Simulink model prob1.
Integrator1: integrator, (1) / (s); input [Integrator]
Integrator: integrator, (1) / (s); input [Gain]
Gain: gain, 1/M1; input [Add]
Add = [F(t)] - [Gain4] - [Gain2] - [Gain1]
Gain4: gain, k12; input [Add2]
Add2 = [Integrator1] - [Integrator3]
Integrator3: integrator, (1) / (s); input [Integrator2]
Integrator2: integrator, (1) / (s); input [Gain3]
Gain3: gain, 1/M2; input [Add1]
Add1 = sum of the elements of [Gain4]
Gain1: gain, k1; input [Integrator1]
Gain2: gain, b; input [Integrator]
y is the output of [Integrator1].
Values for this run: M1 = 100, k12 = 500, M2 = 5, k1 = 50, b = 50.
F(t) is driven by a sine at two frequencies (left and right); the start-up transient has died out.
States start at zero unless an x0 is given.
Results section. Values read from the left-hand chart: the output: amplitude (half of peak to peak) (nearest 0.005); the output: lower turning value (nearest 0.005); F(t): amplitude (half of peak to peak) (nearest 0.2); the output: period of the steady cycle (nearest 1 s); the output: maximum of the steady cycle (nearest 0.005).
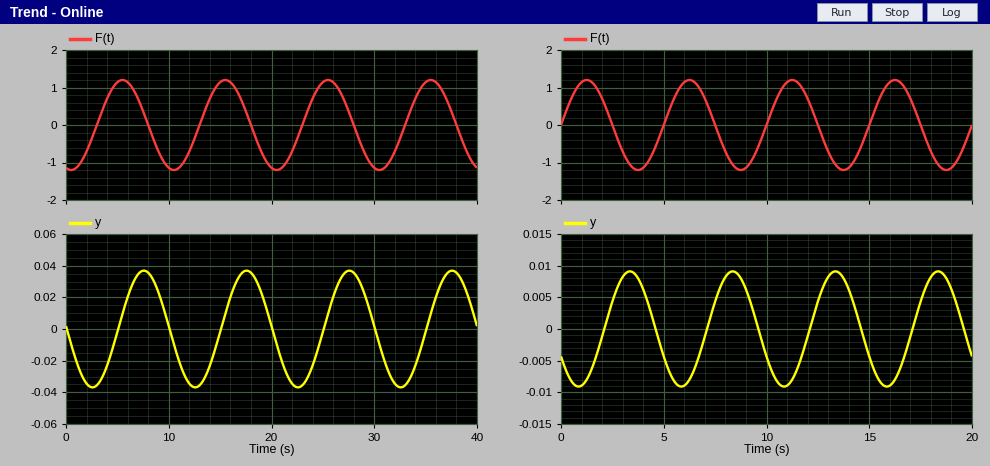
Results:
0.035
-0.035
1.2
10 s
0.035
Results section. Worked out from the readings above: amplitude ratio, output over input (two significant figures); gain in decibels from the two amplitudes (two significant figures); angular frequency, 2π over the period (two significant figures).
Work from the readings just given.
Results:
0.029
-31 dB
0.63 rad/s
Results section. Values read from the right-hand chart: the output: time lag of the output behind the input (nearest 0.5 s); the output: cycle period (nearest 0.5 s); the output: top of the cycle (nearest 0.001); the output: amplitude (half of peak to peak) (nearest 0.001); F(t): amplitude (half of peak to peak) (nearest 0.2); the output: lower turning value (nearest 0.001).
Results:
2.0 s
5.0 s
0.009
0.009
1.2
-0.009
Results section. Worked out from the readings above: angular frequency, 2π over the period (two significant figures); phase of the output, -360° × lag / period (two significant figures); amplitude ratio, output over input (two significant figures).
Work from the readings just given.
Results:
1.3 rad/s
-140°
0.0075
